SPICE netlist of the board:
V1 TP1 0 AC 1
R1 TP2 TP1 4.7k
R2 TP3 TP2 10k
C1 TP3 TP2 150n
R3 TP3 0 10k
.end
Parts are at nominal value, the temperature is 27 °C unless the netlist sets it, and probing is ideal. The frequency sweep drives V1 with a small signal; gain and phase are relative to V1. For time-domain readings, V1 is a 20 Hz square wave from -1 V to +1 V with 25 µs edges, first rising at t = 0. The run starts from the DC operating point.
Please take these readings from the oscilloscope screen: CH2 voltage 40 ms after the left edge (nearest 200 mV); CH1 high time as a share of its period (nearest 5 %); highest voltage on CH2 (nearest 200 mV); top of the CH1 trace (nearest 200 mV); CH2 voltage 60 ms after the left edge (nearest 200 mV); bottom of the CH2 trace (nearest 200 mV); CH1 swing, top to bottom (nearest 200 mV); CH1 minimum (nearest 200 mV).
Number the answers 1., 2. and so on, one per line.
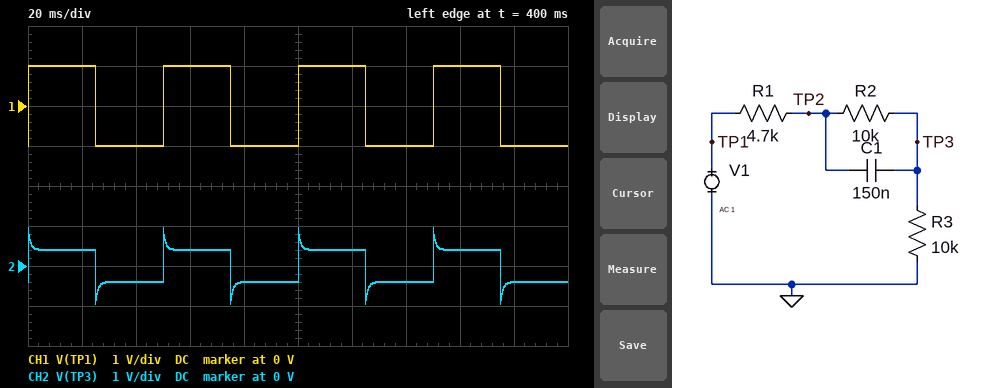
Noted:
1. -400 mV
2. 50 %
3. 1.0 V
4. 1.0 V
5. 400 mV
6. -1.0 V
7. 2.0 V
8. -1.0 V
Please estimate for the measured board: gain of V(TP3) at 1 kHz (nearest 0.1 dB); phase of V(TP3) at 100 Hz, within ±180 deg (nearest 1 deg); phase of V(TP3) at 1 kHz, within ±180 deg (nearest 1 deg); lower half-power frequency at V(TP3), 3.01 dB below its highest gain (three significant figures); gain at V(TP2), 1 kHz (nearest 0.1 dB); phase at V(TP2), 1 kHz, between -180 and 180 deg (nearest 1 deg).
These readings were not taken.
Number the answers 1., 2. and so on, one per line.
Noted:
1. -3.4 dB
2. 14 deg
3. 4 deg
4. 96.3 Hz
5. -3.3 dB
6. -2 deg
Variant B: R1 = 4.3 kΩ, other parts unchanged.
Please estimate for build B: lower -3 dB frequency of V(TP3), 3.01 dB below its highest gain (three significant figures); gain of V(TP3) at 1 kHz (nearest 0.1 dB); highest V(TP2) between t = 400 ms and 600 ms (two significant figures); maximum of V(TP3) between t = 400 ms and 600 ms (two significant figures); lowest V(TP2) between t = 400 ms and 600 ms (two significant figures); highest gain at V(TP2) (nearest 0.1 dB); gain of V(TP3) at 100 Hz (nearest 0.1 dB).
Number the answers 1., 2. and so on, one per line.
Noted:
1. 100 Hz
2. -3.2 dB
3. 820 mV
4. 980 mV
5. -820 mV
6. -1.7 dB
7. -6.1 dB
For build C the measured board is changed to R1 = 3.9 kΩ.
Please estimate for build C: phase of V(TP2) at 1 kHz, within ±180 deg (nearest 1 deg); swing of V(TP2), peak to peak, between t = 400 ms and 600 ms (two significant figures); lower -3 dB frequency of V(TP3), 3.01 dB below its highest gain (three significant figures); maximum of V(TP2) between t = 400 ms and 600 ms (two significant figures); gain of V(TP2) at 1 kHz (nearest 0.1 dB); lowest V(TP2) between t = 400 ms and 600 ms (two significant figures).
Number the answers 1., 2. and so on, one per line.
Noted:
1. -2 deg
2. 1.7 V
3. 104 Hz
4. 840 mV
5. -2.8 dB
6. -840 mV
